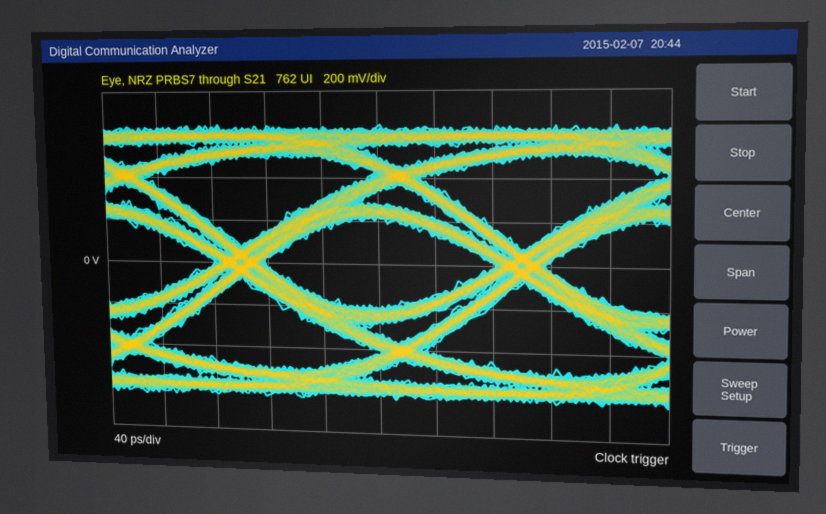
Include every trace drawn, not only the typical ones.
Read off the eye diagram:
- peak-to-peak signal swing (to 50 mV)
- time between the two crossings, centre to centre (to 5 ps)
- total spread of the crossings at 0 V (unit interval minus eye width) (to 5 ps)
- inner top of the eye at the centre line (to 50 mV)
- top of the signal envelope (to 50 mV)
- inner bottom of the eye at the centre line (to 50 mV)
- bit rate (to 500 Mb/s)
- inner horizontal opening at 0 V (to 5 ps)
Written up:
1.30 V
200 ps
35 ps
200 mV
650 mV
-200 mV
5.0 Gb/s
165 ps
